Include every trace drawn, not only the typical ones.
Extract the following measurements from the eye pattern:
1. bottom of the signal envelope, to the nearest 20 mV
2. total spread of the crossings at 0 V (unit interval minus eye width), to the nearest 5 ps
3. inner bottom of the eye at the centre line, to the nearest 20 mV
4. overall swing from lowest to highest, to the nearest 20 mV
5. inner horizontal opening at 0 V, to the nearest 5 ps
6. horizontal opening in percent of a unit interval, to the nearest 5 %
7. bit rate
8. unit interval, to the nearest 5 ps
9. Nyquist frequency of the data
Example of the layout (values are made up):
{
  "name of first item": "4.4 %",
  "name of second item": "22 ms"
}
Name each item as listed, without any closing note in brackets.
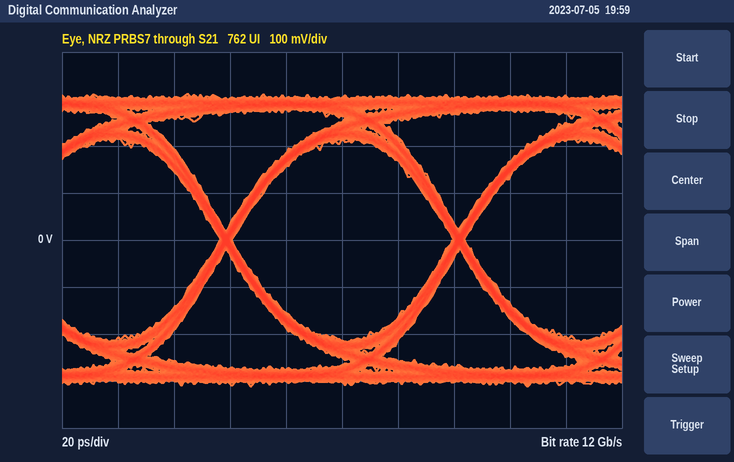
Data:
{
  "bottom of the signal envelope, to the nearest 20 mV": "-320 mV",
  "total spread of the crossings at 0 V (unit interval minus eye width), to the nearest 5 ps": "5 ps",
  "inner bottom of the eye at the centre line, to the nearest 20 mV": "-220 mV",
  "overall swing from lowest to highest, to the nearest 20 mV": "620 mV",
  "inner horizontal opening at 0 V, to the nearest 5 ps": "80 ps",
  "horizontal opening in percent of a unit interval, to the nearest 5 %": "95 %",
  "bit rate": "12 Gb/s",
  "unit interval, to the nearest 5 ps": "85 ps",
  "Nyquist frequency of the data": "6 GHz"
}
